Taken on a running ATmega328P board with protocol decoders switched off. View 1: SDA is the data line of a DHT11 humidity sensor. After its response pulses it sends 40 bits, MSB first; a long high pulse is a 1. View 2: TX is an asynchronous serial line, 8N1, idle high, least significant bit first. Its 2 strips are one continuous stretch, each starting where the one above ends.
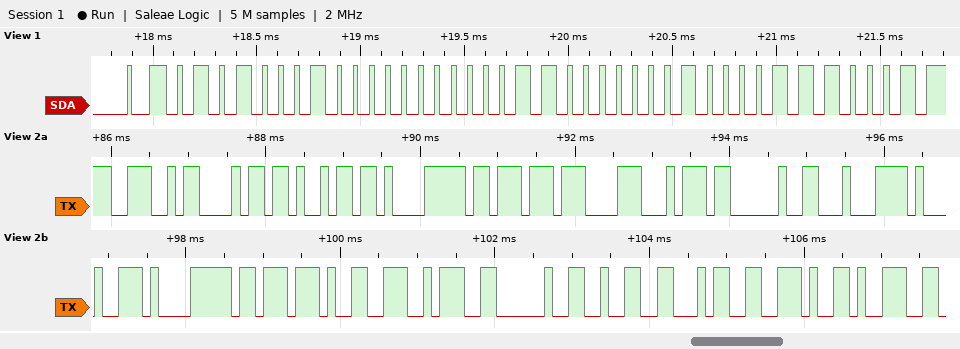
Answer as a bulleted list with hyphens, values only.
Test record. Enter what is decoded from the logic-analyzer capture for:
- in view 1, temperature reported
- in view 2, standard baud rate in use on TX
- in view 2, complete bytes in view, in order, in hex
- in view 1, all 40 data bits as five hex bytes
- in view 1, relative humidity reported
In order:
- 24.8 °C
- 9600 baud
- 4E 68 69 E1 BB 87 74 20 C4 91 E1 BB 99 3A 20 32 34 2E 39
- 51 00 18 08 71
- 81 %
